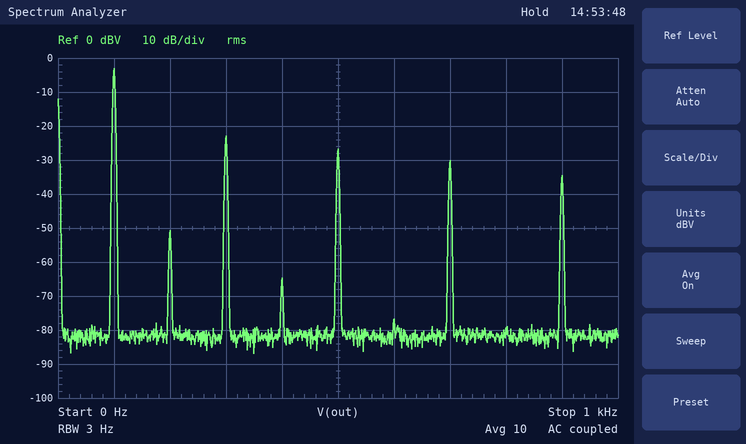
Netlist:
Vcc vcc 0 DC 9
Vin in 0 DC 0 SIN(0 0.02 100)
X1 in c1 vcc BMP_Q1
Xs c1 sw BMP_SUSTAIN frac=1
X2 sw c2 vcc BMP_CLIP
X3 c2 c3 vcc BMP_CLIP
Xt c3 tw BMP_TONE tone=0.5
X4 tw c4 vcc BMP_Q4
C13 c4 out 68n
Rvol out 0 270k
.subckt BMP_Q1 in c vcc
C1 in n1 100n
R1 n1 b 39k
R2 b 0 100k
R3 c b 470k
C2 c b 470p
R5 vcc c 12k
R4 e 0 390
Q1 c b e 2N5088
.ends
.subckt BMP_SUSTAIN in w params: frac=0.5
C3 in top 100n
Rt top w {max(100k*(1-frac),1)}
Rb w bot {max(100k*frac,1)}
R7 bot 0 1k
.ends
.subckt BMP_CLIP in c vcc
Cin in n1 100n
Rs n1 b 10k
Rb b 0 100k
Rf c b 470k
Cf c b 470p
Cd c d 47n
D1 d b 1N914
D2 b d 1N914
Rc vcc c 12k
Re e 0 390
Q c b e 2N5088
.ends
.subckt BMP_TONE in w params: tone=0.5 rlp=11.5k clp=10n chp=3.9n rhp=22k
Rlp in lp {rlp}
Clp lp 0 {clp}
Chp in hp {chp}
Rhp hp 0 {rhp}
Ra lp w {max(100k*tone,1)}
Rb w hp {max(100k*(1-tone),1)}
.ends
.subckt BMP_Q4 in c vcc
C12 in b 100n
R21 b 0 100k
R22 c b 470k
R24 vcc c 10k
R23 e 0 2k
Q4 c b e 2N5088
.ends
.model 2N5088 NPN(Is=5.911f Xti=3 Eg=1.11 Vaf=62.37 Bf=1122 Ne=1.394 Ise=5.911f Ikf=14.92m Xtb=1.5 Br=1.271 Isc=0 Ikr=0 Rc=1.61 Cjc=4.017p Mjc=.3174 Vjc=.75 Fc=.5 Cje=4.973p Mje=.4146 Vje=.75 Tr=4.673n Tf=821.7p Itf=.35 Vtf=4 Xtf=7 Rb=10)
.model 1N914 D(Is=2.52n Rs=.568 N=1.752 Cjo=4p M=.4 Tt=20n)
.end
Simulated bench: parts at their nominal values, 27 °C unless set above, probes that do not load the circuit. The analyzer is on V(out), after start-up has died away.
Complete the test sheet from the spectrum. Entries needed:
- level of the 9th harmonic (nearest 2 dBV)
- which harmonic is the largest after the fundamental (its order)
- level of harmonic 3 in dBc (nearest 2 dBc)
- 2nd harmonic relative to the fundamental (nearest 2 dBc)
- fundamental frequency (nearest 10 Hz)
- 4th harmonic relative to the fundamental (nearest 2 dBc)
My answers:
-34 dBV
3
-20 dBc
-48 dBc
100 Hz
-62 dBc
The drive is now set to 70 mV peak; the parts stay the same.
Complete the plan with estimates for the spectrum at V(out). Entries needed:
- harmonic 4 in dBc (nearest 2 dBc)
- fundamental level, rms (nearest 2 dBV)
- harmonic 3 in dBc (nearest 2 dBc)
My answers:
-52 dBc
0 dBV
-16 dBc
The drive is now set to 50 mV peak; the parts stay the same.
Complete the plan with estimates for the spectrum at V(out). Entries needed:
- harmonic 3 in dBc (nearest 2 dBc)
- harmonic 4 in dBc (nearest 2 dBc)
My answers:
-16 dBc
-54 dBc
